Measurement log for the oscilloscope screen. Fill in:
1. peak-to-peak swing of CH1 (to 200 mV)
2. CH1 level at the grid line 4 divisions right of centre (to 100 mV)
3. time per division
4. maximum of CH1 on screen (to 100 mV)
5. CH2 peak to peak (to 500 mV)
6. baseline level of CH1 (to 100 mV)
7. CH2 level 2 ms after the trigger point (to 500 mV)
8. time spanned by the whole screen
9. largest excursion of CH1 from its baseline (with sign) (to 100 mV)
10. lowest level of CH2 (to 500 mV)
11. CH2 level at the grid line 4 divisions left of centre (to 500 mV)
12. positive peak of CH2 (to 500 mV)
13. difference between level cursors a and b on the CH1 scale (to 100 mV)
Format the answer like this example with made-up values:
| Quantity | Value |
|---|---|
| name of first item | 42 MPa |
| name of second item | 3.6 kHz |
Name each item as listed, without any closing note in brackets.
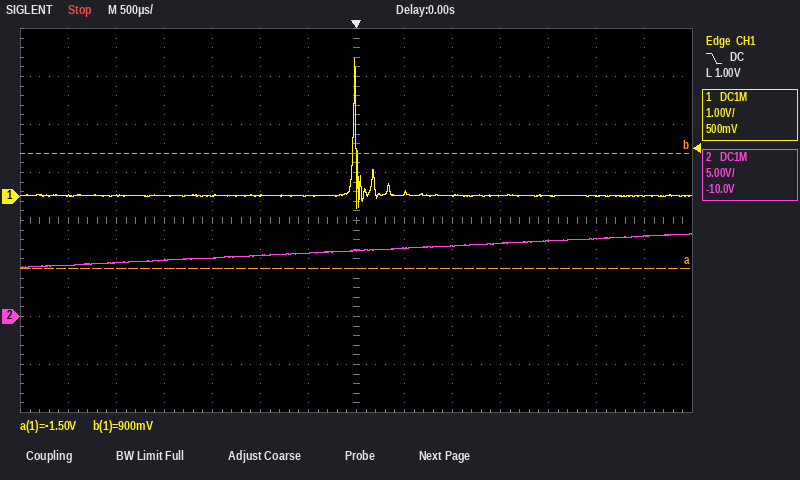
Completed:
| Quantity | Value |
|---|---|
| peak-to-peak swing of CH1 | 3.2 V |
| CH1 level at the grid line 4 divisions right of centre | 0.0 V |
| time per division | 500 µs |
| maximum of CH1 on screen | 2.9 V |
| CH2 peak to peak | 3.5 V |
| baseline level of CH1 | 0.0 V |
| CH2 level 2 ms after the trigger point | 8.0 V |
| time spanned by the whole screen | 7 ms |
| largest excursion of CH1 from its baseline (with sign) | +2.9 V |
| lowest level of CH2 | 5.0 V |
| CH2 level at the grid line 4 divisions left of centre | 6.0 V |
| positive peak of CH2 | 8.5 V |
| difference between level cursors a and b on the CH1 scale | 2.4 V |
